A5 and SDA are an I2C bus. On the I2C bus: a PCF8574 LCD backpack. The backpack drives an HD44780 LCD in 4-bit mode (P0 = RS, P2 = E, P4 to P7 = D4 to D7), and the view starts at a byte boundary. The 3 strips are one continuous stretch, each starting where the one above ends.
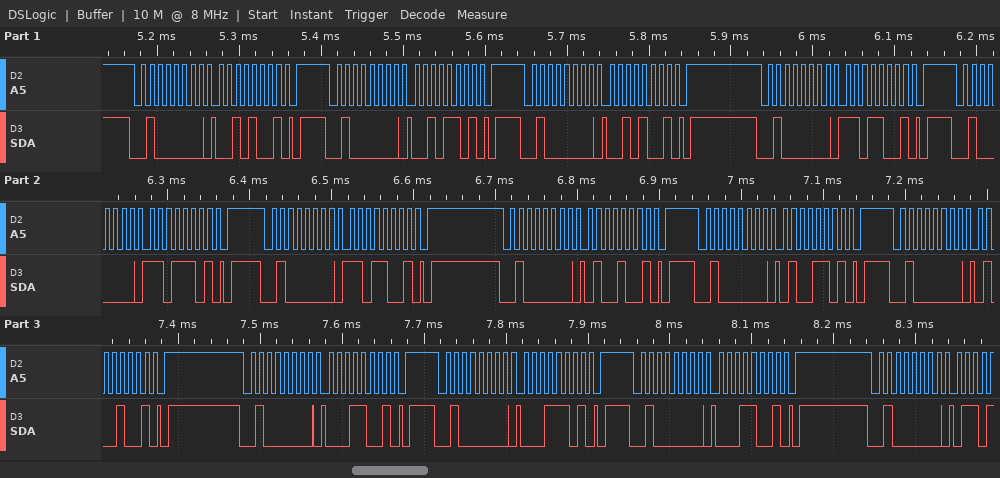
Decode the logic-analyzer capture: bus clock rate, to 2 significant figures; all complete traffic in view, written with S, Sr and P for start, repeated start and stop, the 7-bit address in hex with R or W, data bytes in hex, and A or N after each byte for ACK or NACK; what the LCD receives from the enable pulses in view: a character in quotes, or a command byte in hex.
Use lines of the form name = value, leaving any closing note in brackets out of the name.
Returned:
bus clock rate, to 2 significant figures = 100 kHz
all complete traffic in view, written with S, Sr and P for start, repeated start and stop, the 7-bit address in hex with R or W, data bytes in hex, and A or N after each byte for ACK or NACK = S 20W A 29 A P S 20W A 2D A P S 20W A 29 A P S 20W A D9 A P S 20W A DD A P S 20W A D9 A P S 20W A 49 A P S 20W A 4D A P S 20W A 49 A P S 20W A 19 A P S 20W A 1D A P S 20W A 19 A P S 20W A
what the LCD receives from the enable pulses in view: a character in quotes, or a command byte in hex = '-' 'A'
